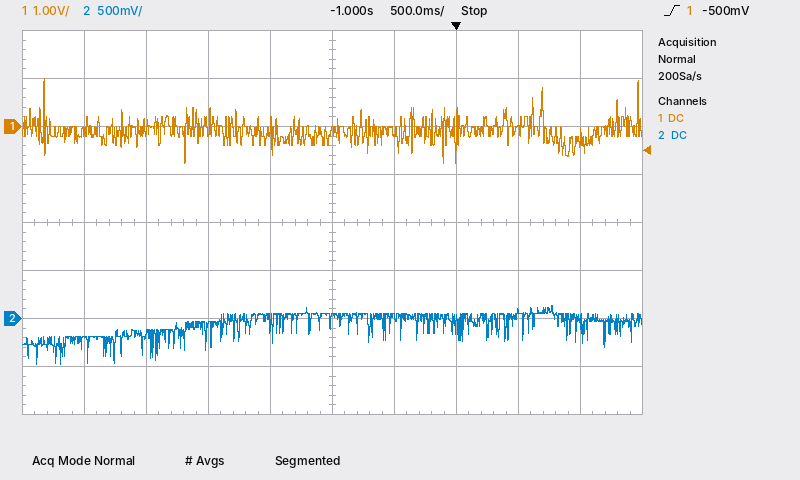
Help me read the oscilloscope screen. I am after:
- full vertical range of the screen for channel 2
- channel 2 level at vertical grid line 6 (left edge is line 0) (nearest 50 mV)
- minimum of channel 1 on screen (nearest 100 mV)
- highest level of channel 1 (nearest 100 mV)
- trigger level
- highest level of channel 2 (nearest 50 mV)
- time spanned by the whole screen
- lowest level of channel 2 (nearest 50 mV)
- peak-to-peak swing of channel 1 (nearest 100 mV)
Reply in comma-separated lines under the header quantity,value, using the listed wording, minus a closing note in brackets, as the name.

quantity,value
full vertical range of the screen for channel 2,4 V
channel 2 level at vertical grid line 6 (left edge is line 0),0 mV
minimum of channel 1 on screen,-800 mV
highest level of channel 1,1.0 V
trigger level,-500 mV
highest level of channel 2,150 mV
time spanned by the whole screen,5 s
lowest level of channel 2,-500 mV
peak-to-peak swing of channel 1,1.8 V
